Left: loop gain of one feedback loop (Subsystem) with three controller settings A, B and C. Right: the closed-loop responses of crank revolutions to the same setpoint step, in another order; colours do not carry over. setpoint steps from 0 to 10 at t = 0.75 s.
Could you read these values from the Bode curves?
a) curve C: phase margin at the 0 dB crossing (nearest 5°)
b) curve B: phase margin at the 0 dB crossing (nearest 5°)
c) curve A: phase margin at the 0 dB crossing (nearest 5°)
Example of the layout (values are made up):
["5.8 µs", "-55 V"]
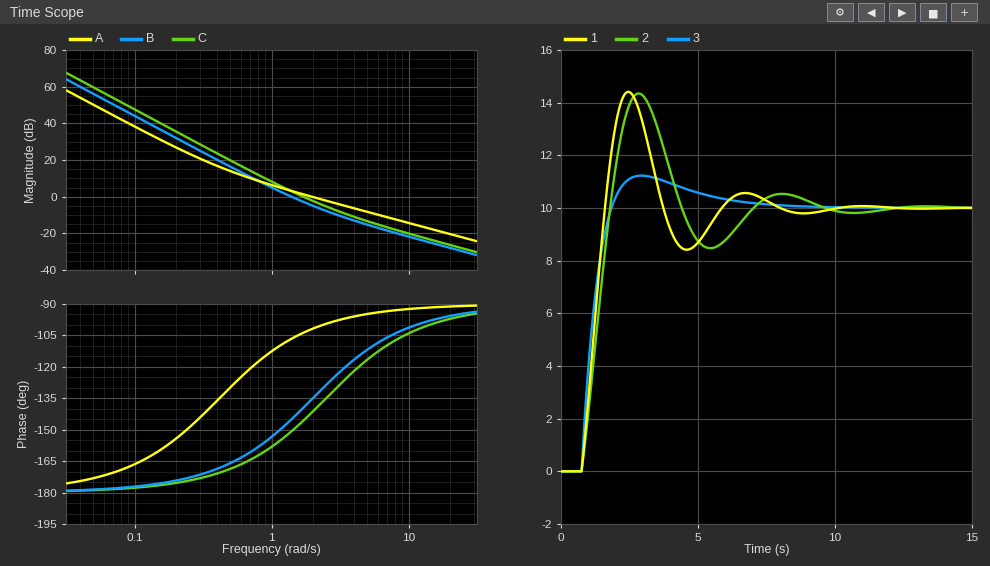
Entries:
["35°", "35°", "80°"]
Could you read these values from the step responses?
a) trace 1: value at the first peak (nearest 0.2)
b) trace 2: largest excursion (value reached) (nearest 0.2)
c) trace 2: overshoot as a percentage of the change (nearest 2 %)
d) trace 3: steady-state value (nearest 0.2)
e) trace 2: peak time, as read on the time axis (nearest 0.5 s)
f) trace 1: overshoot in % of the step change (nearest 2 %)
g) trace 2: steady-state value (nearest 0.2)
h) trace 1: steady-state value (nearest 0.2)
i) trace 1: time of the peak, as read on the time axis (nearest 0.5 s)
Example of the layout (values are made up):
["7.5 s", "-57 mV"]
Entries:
["14.4", "14.4", "44 %", "10.0", "3.0 s", "44 %", "10.0", "10.0", "2.5 s"]
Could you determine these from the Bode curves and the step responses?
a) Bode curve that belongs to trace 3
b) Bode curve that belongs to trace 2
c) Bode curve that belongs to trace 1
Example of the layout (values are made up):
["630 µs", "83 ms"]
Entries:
["A", "B", "C"]
